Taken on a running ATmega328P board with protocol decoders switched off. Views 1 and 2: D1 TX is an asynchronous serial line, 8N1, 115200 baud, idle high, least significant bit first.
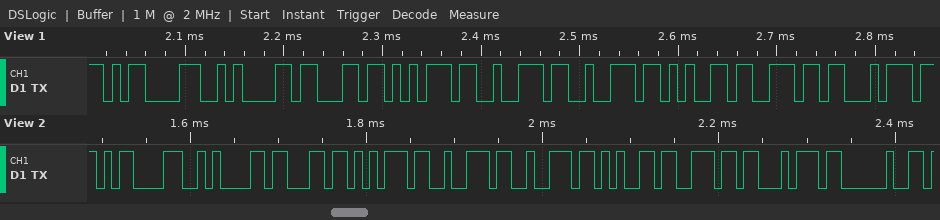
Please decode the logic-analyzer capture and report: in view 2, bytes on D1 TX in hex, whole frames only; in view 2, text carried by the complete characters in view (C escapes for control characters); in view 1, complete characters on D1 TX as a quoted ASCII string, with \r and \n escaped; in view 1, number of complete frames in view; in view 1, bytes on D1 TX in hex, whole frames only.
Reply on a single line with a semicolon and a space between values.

0D 0A 63 75 72 72 65 6E 74 20; "\r\ncurrent "; "\r\ncurrent"; 9; 0D 0A 63 75 72 72 65 6E 74
